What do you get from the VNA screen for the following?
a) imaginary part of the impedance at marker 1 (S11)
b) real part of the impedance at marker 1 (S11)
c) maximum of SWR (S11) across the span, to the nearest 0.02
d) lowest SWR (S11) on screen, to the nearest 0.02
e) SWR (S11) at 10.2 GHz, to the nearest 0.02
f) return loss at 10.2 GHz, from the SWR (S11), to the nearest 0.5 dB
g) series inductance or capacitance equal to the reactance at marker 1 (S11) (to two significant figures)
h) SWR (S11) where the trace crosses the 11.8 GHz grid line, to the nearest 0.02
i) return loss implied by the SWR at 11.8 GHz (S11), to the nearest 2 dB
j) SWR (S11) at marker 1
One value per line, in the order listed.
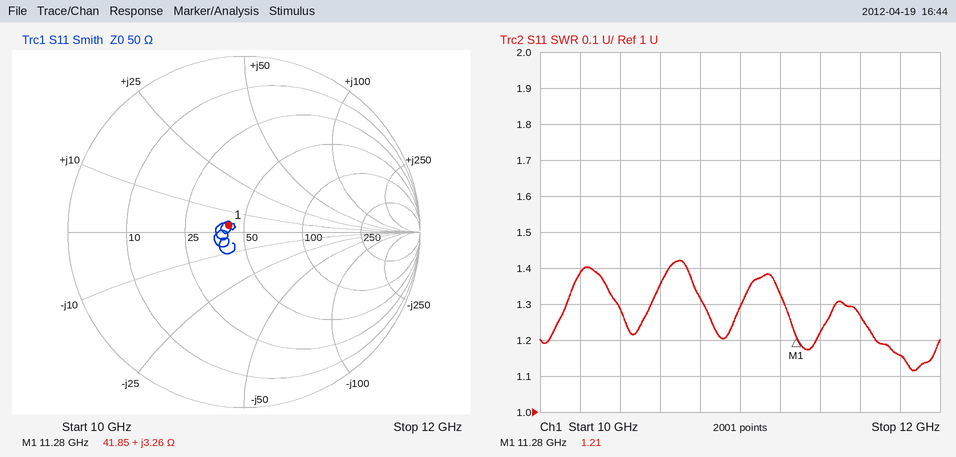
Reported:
+3.26 Ω
41.85 Ω
1.42
1.12
1.38
16.0 dB
46 pH
1.16
22 dB
1.21
